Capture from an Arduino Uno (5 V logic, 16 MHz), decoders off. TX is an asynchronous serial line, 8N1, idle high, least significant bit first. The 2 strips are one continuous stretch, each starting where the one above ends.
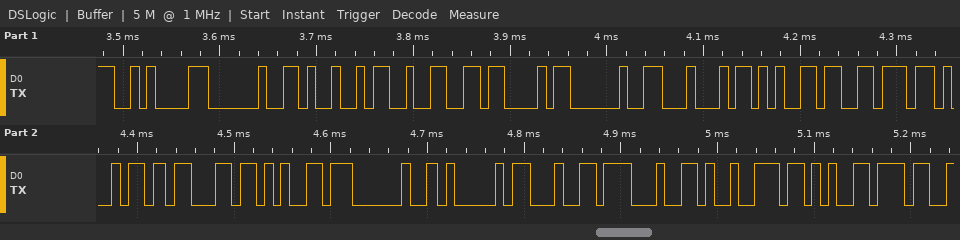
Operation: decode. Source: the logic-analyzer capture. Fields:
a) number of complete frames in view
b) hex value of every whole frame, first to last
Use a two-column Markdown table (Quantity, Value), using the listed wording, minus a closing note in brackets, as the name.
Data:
| Quantity | Value |
|---|---|
| number of complete frames in view | 18 |
| hex value of every whole frame, first to last | 0x0A 0x20 0x49 0x32 0x43 0x20 0x44 0x65 0x76 0x69 0x63 0x65 0x20 0x41 0x64 0x64 0x72 0x65 |
